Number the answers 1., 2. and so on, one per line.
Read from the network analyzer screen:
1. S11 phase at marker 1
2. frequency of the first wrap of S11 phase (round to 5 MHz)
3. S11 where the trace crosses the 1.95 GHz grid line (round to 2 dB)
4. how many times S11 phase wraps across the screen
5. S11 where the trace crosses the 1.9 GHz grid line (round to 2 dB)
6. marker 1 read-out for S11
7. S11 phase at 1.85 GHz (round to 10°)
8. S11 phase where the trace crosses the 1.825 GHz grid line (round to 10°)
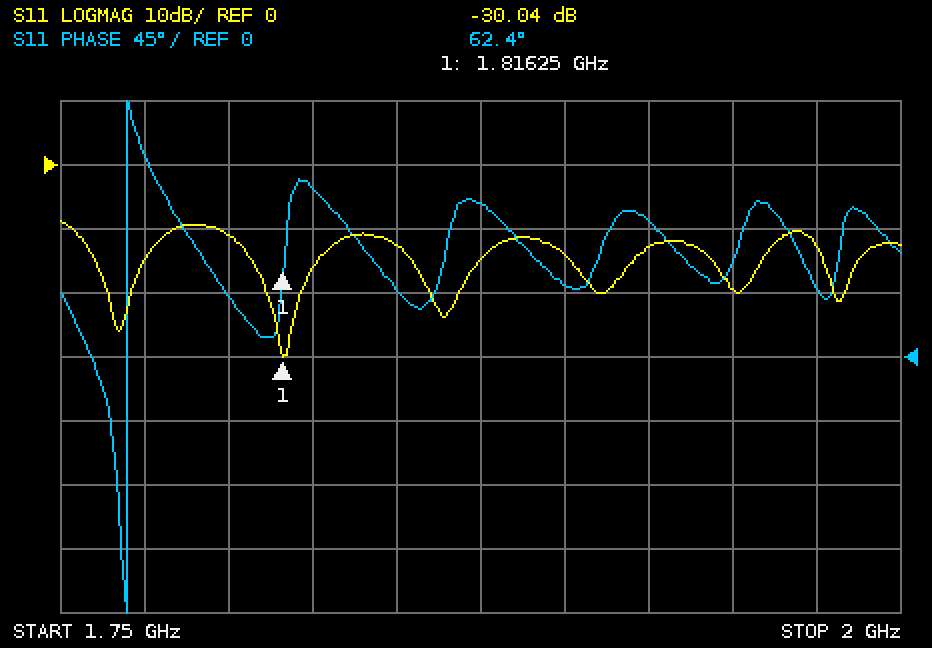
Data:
1. 62.4°
2. 1.770 GHz
3. -20 dB
4. 1
5. -14 dB
6. -30.04 dB
7. 50°
8. 120°
